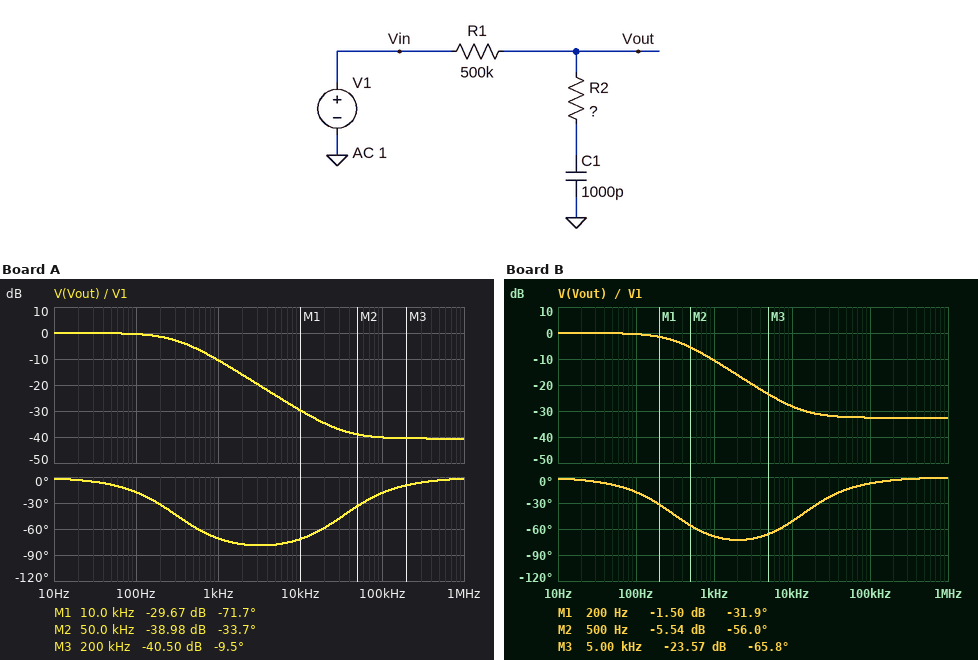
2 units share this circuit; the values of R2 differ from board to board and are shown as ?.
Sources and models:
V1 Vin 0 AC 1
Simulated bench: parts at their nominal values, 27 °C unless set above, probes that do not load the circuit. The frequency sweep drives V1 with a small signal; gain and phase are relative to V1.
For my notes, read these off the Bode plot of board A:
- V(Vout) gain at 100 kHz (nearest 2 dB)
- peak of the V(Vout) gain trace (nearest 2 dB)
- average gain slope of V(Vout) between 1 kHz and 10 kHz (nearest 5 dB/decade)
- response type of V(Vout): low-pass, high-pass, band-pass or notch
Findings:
-40 dB
0 dB
-20 dB/decade
low-pass
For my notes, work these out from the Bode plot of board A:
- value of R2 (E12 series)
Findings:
4.7 kΩ
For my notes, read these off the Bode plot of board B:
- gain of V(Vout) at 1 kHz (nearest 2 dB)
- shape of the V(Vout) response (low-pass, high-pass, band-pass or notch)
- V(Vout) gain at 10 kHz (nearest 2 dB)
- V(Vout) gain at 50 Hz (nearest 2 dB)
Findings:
-10 dB
low-pass
-28 dB
0 dB
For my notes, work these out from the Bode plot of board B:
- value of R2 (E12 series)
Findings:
12 kΩ
